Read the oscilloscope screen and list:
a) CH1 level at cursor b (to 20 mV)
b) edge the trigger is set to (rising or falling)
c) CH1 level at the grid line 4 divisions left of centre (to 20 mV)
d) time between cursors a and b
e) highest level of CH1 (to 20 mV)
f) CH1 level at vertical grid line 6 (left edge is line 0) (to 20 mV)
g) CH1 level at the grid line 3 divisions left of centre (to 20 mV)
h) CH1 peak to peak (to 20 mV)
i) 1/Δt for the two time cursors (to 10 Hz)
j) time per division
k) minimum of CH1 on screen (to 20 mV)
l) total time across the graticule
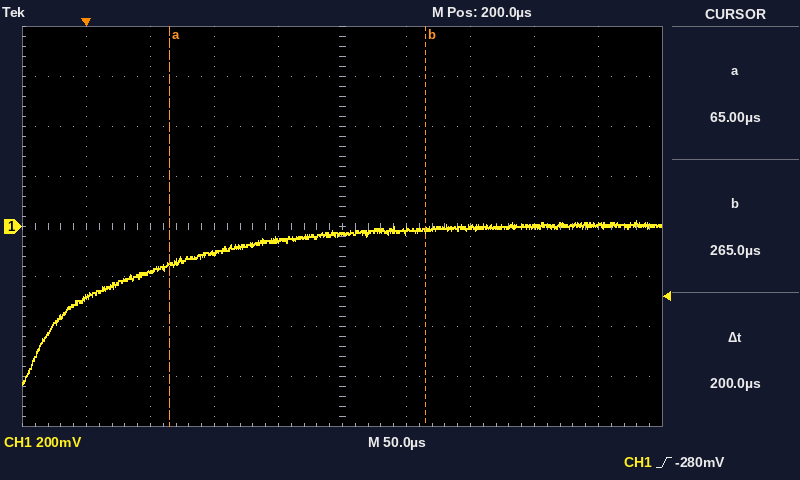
-20 mV
rising
-280 mV
200 µs
20 mV
-20 mV
-180 mV
660 mV
5.00 kHz
50 µs
-640 mV
500 µs
